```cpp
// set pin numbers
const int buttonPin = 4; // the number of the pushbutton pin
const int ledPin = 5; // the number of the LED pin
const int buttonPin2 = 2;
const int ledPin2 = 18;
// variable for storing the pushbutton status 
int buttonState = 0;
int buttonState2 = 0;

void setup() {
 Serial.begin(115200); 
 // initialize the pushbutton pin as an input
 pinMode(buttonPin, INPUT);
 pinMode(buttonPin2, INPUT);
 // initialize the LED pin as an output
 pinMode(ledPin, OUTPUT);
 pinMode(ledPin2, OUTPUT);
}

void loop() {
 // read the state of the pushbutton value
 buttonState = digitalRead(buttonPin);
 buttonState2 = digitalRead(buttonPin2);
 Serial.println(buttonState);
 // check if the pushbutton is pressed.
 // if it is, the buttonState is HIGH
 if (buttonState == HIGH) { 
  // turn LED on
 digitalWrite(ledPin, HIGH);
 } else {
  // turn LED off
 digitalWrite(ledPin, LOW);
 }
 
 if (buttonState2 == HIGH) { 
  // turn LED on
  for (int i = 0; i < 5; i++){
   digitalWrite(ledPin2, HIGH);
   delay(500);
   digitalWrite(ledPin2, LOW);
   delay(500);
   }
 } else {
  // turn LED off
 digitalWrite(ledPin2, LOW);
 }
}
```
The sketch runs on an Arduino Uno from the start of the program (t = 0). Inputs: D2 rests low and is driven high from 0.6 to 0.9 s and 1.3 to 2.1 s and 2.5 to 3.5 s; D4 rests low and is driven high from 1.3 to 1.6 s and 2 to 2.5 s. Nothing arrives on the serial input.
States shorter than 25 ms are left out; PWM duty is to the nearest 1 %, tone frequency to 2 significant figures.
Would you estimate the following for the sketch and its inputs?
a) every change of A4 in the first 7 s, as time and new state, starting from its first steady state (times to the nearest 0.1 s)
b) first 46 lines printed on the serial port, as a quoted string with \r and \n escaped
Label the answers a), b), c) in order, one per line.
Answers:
a) 0 s low; 0.6 s high; 1.1 s low; 1.6 s high; 2.1 s low; 2.6 s high; 3.1 s low; 3.6 s high; 4.1 s low; 4.6 s high; 5.1 s low
b) "0\r\n0\r\n0\r\n0\r\n0\r\n0\r\n0\r\n0\r\n0\r\n0\r\n0\r\n0\r\n0\r\n0\r\n0\r\n0\r\n0\r\n0\r\n0\r\n0\r\n0\r\n0\r\n0\r\n0\r\n0\r\n0\r\n0\r\n0\r\n0\r\n0\r\n0\r\n0\r\n0\r\n0\r\n0\r\n0\r\n0\r\n0\r\n0\r\n0\r\n0\r\n0\r\n0\r\n0\r\n0\r\n0\r\n"
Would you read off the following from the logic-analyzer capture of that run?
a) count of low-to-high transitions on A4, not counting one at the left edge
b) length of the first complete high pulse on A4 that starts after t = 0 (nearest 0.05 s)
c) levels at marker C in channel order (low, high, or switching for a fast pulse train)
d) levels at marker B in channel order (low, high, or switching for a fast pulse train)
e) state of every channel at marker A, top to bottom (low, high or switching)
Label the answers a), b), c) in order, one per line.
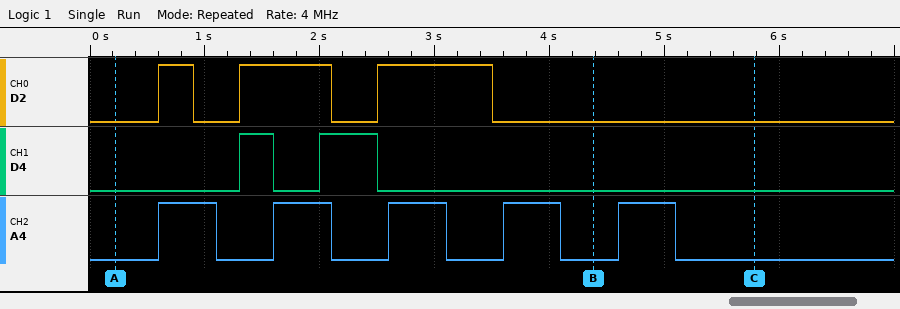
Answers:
a) 5
b) 0.50 s
c) D2 low, D4 low, A4 low
d) D2 low, D4 low, A4 low
e) D2 low, D4 low, A4 low
